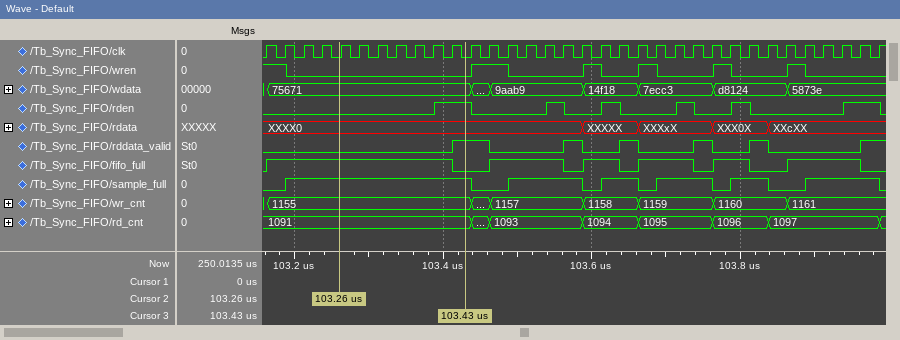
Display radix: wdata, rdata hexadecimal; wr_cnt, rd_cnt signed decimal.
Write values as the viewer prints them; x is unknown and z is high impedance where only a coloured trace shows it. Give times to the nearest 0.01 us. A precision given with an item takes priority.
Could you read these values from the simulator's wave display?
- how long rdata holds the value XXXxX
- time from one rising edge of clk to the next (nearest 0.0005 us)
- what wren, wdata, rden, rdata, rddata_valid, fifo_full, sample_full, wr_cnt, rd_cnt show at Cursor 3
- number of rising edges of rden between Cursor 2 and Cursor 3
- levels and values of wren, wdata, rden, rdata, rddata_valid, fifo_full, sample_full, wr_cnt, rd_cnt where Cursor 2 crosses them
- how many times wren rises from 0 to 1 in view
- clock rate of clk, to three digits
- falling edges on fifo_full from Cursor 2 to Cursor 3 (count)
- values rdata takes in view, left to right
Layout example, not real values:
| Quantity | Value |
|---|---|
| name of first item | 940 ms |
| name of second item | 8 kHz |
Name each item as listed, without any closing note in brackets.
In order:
| Quantity | Value |
|---|---|
| how long rdata holds the value XXXxX | 0.1 us |
| time from one rising edge of clk to the next | 0.025 us |
| what wren, wdata, rden, rdata, rddata_valid, fifo_full, sample_full, wr_cnt, rd_cnt show at Cursor 3 | wren=0, wdata=75671, rden=1, rdata=XXXX0, rddata_valid=1, fifo_full=0, sample_full=1, wr_cnt=1155, rd_cnt=1091 |
| number of rising edges of rden between Cursor 2 and Cursor 3 | 1 |
| levels and values of wren, wdata, rden, rdata, rddata_valid, fifo_full, sample_full, wr_cnt, rd_cnt where Cursor 2 crosses them | wren=0, wdata=75671, rden=0, rdata=XXXX0, rddata_valid=0, fifo_full=1, sample_full=1, wr_cnt=1155, rd_cnt=1091 |
| how many times wren rises from 0 to 1 in view | 5 |
| clock rate of clk, to three digits | 40.0 MHz |
| falling edges on fifo_full from Cursor 2 to Cursor 3 | 1 |
| values rdata takes in view, left to right | XXXX0, XXXXX, XXXxX, XXX0X, XXcXX |
